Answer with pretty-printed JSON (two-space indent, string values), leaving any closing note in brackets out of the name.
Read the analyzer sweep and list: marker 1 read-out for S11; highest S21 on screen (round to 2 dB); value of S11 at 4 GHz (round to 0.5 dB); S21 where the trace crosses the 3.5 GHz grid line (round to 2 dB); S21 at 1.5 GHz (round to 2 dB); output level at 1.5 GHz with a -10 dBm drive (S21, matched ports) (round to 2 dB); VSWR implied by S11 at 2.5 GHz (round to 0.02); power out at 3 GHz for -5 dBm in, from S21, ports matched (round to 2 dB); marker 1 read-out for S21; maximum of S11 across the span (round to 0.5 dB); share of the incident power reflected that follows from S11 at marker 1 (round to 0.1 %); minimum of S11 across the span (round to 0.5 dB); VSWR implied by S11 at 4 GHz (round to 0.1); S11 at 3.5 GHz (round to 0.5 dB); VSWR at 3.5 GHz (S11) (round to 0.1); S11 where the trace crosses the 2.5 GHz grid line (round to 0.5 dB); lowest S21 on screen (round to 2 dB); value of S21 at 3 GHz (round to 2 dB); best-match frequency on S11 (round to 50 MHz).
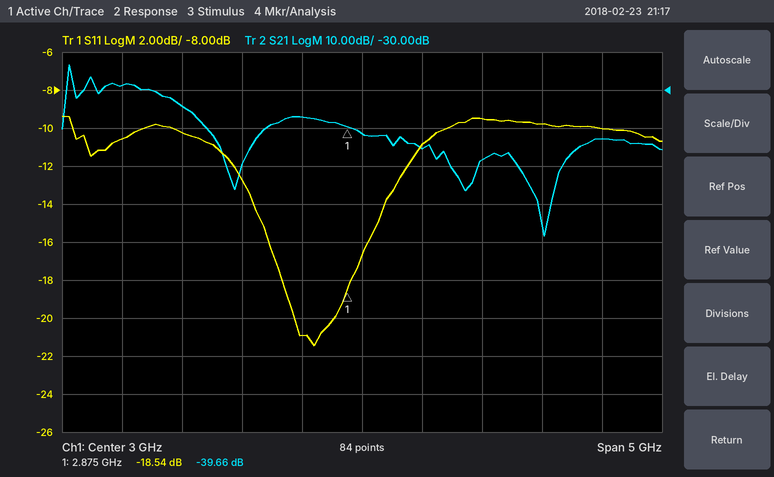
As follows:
{
  "marker 1 read-out for S11": "-18.54 dB",
  "highest S21 on screen": "-24 dB",
  "value of S11 at 4 GHz": "-9.5 dB",
  "S21 where the trace crosses the 3.5 GHz grid line": "-46 dB",
  "S21 at 1.5 GHz": "-34 dB",
  "output level at 1.5 GHz with a -10 dBm drive (S21, matched ports)": "-44 dBm",
  "VSWR implied by S11 at 2.5 GHz": "1.20",
  "power out at 3 GHz for -5 dBm in, from S21, ports matched": "-46 dBm",
  "marker 1 read-out for S21": "-39.66 dB",
  "maximum of S11 across the span": "-9.5 dB",
  "share of the incident power reflected that follows from S11 at marker 1": "1.4 %",
  "minimum of S11 across the span": "-21.5 dB",
  "VSWR implied by S11 at 4 GHz": "2.0",
  "S11 at 3.5 GHz": "-11.0 dB",
  "VSWR at 3.5 GHz (S11)": "1.8",
  "S11 where the trace crosses the 2.5 GHz grid line": "-21.0 dB",
  "lowest S21 on screen": "-68 dB",
  "value of S21 at 3 GHz": "-42 dB",
  "best-match frequency on S11": "2.60 GHz"
}
